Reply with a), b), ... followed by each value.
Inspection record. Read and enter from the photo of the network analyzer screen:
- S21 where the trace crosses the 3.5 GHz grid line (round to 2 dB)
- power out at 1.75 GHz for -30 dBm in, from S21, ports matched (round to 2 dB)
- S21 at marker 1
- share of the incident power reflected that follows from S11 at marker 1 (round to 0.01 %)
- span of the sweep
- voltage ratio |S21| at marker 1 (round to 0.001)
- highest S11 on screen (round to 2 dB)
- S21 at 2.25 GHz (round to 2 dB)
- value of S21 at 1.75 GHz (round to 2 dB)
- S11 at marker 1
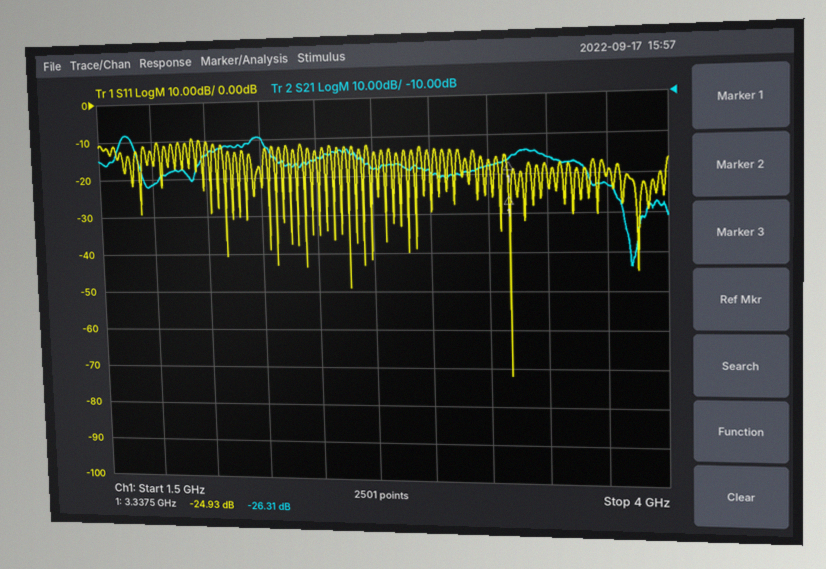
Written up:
a) -26 dB
b) -62 dBm
c) -26.31 dB
d) 0.32 %
e) 2.5 GHz
f) 0.048
g) -10 dB
h) -20 dB
i) -32 dB
j) -24.93 dB
